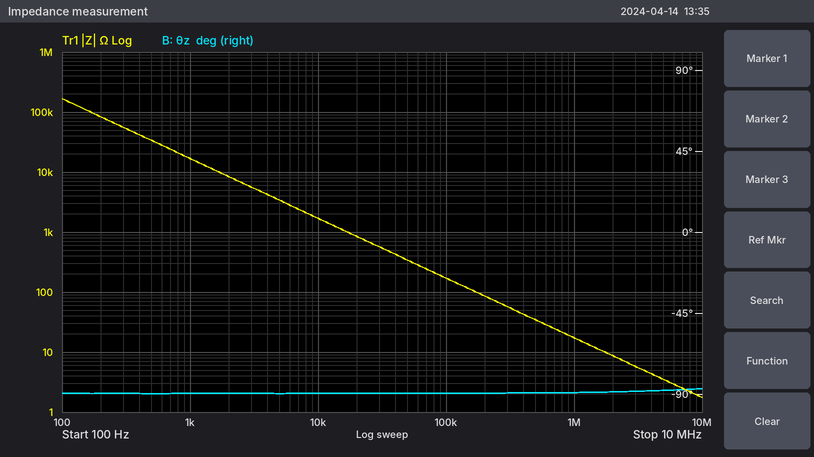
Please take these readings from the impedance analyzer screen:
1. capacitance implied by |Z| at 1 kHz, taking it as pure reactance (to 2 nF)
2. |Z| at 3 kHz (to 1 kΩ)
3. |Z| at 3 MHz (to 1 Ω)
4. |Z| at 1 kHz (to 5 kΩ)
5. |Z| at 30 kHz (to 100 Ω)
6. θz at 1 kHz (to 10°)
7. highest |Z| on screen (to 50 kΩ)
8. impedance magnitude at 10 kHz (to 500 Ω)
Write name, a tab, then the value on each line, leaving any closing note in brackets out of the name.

capacitance implied by |Z| at 1 kHz, taking it as pure reactance	10 nF
|Z| at 3 kHz	6 kΩ
|Z| at 3 MHz	6 Ω
|Z| at 1 kHz	15 kΩ
|Z| at 30 kHz	600 Ω
θz at 1 kHz	-90°
highest |Z| on screen	150 kΩ
impedance magnitude at 10 kHz	1.5 kΩ
